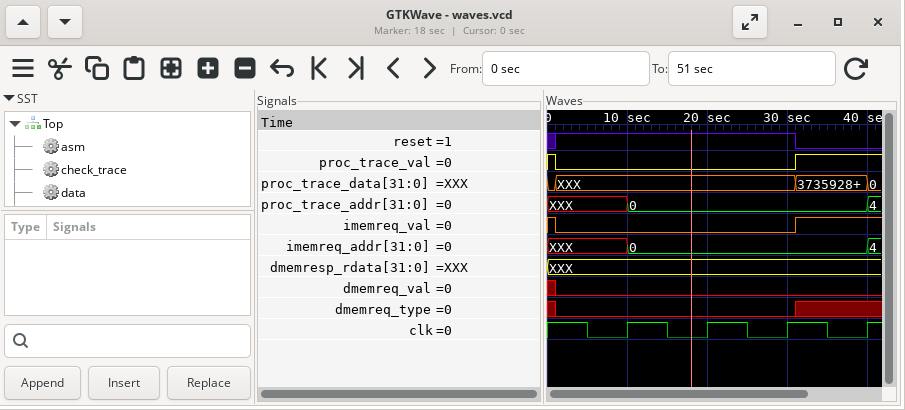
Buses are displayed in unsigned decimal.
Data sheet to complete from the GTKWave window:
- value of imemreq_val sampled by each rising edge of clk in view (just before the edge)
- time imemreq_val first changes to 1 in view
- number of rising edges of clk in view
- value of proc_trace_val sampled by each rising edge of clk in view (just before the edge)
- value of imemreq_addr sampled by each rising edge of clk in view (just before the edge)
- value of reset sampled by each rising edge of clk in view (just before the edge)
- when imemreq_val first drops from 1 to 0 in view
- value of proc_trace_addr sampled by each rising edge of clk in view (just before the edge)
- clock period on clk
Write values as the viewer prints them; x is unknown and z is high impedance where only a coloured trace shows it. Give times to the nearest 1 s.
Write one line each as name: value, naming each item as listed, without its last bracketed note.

value of imemreq_val sampled by each rising edge of clk in view: 0 0 0 1
time imemreq_val first changes to 1 in view: 31 s
number of rising edges of clk in view: 4
value of proc_trace_val sampled by each rising edge of clk in view: 0 0 0 1
value of imemreq_addr sampled by each rising edge of clk in view: XXX, 0, 0, 0
value of reset sampled by each rising edge of clk in view: 1 1 1 0
when imemreq_val first drops from 1 to 0 in view: 1 s
value of proc_trace_addr sampled by each rising edge of clk in view: XXX, 0, 0, 0
clock period on clk: 10 s
